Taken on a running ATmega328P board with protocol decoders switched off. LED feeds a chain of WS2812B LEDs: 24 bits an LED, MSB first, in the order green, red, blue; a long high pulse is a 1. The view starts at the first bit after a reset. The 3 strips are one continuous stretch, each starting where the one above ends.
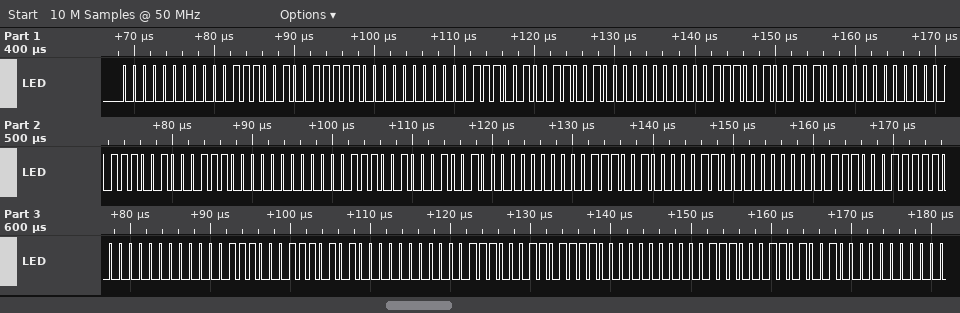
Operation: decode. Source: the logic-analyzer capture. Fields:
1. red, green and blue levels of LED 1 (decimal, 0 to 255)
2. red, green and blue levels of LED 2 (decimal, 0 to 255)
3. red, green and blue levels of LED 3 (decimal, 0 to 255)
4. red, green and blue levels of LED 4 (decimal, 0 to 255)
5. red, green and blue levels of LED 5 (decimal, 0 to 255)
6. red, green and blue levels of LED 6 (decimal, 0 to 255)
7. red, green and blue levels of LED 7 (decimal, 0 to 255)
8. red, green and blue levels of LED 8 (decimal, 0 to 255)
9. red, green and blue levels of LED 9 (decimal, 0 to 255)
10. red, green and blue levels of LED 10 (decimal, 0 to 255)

28, 0, 159
28, 0, 153
28, 0, 148
28, 0, 142
28, 0, 137
28, 0, 131
28, 0, 124
28, 0, 117
28, 0, 111
28, 0, 105
